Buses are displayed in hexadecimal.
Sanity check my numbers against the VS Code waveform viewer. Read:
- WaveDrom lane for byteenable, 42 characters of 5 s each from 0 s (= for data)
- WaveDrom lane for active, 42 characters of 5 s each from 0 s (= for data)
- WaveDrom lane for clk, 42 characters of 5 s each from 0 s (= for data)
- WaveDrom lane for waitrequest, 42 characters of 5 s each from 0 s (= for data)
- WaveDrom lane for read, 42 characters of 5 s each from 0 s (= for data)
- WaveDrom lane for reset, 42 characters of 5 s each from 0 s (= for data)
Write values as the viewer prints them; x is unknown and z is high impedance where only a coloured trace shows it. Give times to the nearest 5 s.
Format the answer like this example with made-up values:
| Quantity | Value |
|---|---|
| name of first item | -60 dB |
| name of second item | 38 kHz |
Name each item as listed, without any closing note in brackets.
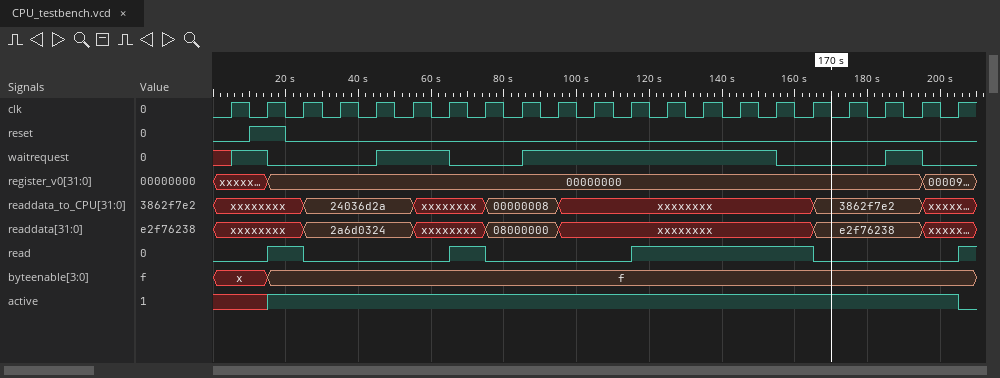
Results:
| Quantity | Value |
|---|---|
| WaveDrom lane for byteenable, 42 characters of 5 s each from 0 s | {name: 'byteenable', wave: 'x..=......................................', data: 'f'} |
| WaveDrom lane for active, 42 characters of 5 s each from 0 s | {name: 'active', wave: 'x..1.....................................0'} |
| WaveDrom lane for clk, 42 characters of 5 s each from 0 s | {name: 'clk', wave: '010101010101010101010101010101010101010101'} |
| WaveDrom lane for waitrequest, 42 characters of 5 s each from 0 s | {name: 'waitrequest', wave: 'x1.0.....1...0...1.............0.....1.0..'} |
| WaveDrom lane for read, 42 characters of 5 s each from 0 s | {name: 'read', wave: '0..1.0.......1.0.......1.........0.......1'} |
| WaveDrom lane for reset, 42 characters of 5 s each from 0 s | {name: 'reset', wave: '0.1.0.....................................'} |
